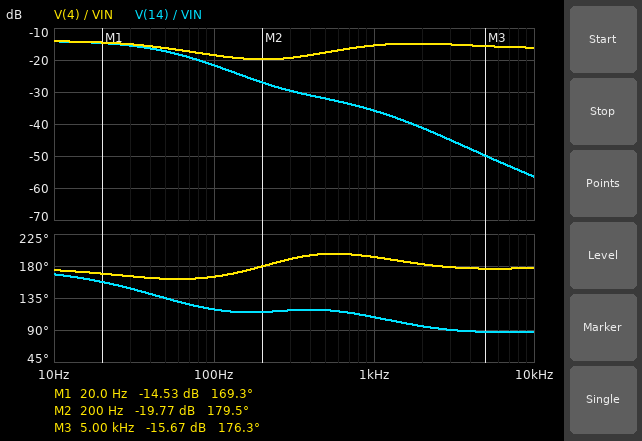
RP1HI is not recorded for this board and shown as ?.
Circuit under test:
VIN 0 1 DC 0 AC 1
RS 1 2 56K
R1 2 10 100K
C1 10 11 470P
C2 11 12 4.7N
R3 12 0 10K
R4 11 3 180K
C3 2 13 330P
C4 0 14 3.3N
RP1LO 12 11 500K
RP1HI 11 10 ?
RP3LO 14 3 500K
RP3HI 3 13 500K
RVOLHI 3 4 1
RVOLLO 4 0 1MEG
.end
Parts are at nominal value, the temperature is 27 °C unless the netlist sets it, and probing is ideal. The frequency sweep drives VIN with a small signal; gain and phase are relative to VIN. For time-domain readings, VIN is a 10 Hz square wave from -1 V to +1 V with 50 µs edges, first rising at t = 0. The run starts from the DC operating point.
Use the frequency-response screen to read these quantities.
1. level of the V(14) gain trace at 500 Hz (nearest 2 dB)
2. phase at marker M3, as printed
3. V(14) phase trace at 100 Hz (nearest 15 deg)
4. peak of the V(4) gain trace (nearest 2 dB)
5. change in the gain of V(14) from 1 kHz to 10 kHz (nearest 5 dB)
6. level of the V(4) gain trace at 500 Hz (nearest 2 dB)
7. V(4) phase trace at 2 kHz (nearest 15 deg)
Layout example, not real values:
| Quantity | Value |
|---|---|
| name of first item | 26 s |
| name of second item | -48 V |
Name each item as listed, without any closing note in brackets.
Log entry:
| Quantity | Value |
|---|---|
| level of the V(14) gain trace at 500 Hz | -32 dB |
| phase at marker M3, as printed | 176.3 deg |
| V(14) phase trace at 100 Hz | 120 deg |
| peak of the V(4) gain trace | -14 dB |
| change in the gain of V(14) from 1 kHz to 10 kHz | -20 dB |
| level of the V(4) gain trace at 500 Hz | -18 dB |
| V(4) phase trace at 2 kHz | 180 deg |
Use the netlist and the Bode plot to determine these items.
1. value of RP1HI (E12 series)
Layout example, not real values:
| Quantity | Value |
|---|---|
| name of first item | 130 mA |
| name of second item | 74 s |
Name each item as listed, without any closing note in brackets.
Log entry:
| Quantity | Value |
|---|---|
| value of RP1HI | 1 MΩ |
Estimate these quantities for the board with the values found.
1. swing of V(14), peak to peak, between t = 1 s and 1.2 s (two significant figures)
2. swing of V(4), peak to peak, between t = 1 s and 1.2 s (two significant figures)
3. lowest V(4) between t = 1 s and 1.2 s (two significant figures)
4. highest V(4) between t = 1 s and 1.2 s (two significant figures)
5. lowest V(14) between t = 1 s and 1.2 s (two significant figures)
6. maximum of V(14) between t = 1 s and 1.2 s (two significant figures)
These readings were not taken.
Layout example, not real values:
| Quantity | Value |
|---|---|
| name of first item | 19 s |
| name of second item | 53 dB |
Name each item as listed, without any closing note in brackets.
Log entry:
| Quantity | Value |
|---|---|
| swing of V(14), peak to peak, between t = 1 s and 1.2 s | 400 mV |
| swing of V(4), peak to peak, between t = 1 s and 1.2 s | 400 mV |
| lowest V(4) between t = 1 s and 1.2 s | -200 mV |
| highest V(4) between t = 1 s and 1.2 s | 200 mV |
| lowest V(14) between t = 1 s and 1.2 s | -200 mV |
| maximum of V(14) between t = 1 s and 1.2 s | 200 mV |
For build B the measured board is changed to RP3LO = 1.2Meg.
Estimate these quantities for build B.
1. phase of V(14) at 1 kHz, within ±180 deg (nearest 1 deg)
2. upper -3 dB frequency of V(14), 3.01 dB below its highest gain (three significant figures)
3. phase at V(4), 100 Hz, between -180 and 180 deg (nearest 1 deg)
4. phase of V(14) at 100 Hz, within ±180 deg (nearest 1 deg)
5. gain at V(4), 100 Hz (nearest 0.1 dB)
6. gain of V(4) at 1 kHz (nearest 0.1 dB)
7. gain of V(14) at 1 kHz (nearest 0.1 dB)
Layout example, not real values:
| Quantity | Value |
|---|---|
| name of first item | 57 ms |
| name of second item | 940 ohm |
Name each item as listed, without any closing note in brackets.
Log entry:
| Quantity | Value |
|---|---|
| phase of V(14) at 1 kHz, within ±180 deg | 104 deg |
| upper -3 dB frequency of V(14), 3.01 dB below its highest gain | 28.8 Hz |
| phase at V(4), 100 Hz, between -180 and 180 deg | 171 deg |
| phase of V(14) at 100 Hz, within ±180 deg | 103 deg |
| gain at V(4), 100 Hz | -17.4 dB |
| gain of V(4) at 1 kHz | -14.3 dB |
| gain of V(14) at 1 kHz | -42.2 dB |
